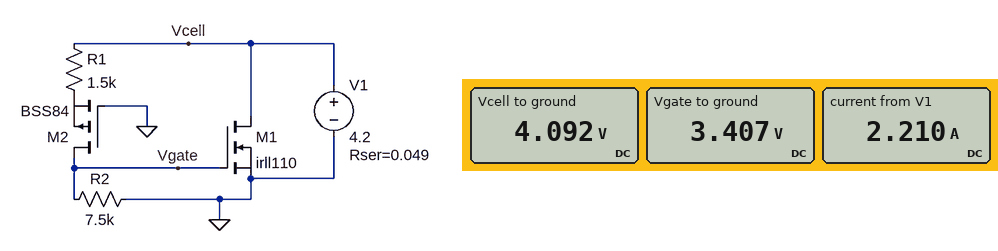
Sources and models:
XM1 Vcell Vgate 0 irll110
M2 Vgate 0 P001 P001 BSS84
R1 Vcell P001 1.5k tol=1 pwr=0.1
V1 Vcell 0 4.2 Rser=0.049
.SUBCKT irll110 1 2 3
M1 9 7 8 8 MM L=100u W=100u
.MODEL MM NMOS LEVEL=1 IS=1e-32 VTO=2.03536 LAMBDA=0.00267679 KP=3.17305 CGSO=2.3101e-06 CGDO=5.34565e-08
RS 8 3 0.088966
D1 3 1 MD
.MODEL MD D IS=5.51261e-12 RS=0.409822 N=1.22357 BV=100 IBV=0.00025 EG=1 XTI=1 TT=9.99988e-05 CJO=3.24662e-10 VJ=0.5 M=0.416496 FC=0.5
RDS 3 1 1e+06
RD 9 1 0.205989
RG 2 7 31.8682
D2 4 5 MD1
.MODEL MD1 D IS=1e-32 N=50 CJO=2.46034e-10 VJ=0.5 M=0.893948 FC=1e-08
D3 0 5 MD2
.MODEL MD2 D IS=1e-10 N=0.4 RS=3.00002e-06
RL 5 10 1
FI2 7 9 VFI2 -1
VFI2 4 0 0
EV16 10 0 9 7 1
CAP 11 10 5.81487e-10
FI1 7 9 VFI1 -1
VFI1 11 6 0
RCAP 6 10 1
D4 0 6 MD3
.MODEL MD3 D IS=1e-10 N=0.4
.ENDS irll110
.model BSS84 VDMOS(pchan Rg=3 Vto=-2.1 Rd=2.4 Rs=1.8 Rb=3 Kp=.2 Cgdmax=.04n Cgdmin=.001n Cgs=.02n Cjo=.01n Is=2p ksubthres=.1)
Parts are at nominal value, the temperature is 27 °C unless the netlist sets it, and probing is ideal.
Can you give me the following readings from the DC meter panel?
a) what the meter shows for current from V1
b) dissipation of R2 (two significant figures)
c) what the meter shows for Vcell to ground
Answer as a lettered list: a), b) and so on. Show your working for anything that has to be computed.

a) 2.210 A
b) (3.407 V)^2 / 7.5 kΩ = 1.5 mW
c) 4.092 V
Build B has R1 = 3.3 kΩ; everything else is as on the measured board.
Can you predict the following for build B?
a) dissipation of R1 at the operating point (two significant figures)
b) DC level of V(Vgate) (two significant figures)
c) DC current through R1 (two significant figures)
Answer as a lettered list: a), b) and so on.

a) 490 µW
b) 2.9 V
c) 380 µA
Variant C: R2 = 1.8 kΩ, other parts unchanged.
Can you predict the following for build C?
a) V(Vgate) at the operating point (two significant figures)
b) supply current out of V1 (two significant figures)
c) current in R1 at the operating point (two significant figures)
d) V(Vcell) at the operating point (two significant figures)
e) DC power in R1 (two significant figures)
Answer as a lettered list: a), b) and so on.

a) 2.3 V
b) 83 mA
c) 1.3 mA
d) 4.2 V
e) 2.4 mW
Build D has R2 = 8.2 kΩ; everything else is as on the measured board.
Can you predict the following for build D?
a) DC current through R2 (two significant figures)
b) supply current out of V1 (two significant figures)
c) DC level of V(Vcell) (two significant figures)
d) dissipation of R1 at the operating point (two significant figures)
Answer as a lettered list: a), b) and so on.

a) 420 µA
b) 2.3 A
c) 4.1 V
d) 270 µW
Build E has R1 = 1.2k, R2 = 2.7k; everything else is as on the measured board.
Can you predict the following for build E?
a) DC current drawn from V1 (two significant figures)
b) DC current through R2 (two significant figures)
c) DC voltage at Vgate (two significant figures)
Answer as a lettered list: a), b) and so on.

a) 910 mA
b) 1.1 mA
c) 2.9 V
